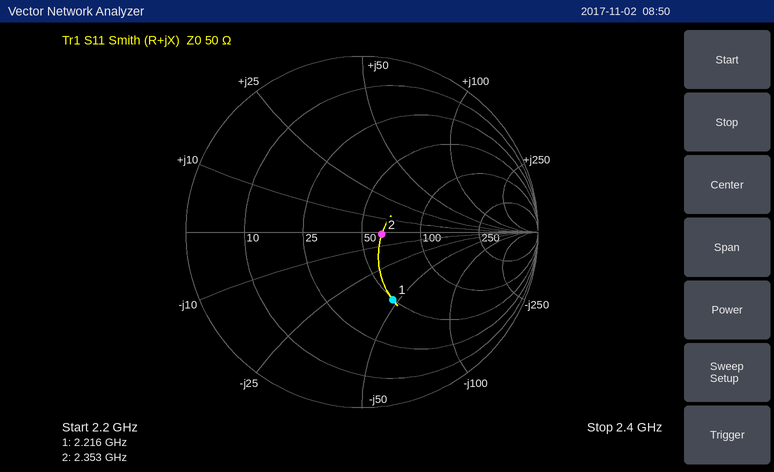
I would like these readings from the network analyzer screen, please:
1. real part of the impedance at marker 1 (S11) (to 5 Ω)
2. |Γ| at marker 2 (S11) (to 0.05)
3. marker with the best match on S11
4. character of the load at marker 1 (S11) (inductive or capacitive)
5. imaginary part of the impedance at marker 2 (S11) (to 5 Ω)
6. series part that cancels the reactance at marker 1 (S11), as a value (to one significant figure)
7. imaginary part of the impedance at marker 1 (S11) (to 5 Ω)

50 Ω
0.10
marker 2
capacitive
0 Ω
3 nH
-45 Ω
